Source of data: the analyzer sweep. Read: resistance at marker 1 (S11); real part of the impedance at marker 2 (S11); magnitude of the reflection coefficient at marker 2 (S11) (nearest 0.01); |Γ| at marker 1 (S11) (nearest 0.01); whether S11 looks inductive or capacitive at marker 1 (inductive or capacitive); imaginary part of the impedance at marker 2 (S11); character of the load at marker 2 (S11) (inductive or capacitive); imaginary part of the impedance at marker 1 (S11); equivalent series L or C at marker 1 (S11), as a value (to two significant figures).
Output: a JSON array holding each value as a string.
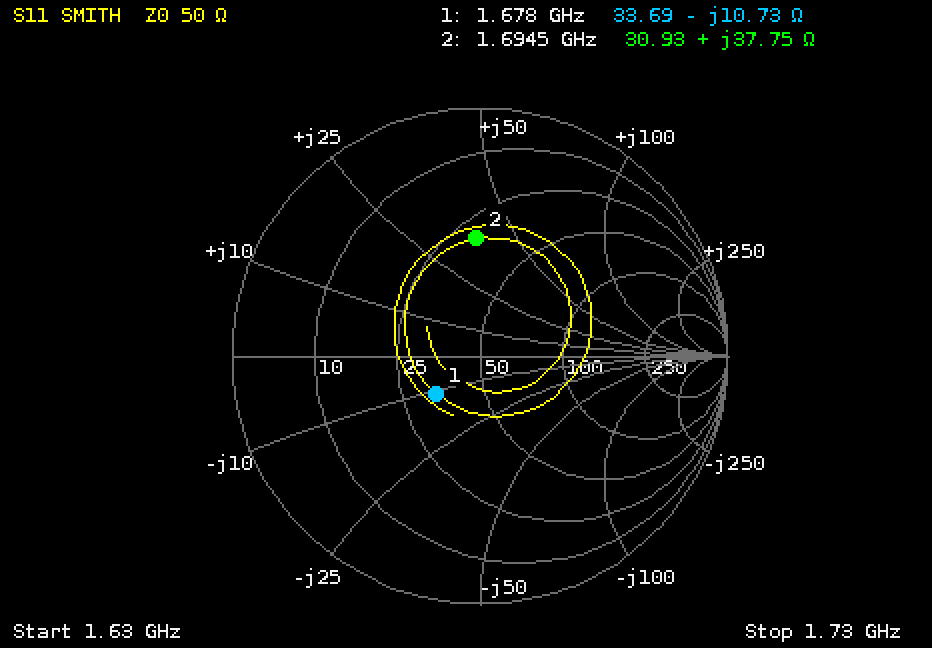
["33.69 Ω", "30.93 Ω", "0.47", "0.23", "capacitive", "+37.75 Ω", "inductive", "-10.73 Ω", "8.8 pF"]
